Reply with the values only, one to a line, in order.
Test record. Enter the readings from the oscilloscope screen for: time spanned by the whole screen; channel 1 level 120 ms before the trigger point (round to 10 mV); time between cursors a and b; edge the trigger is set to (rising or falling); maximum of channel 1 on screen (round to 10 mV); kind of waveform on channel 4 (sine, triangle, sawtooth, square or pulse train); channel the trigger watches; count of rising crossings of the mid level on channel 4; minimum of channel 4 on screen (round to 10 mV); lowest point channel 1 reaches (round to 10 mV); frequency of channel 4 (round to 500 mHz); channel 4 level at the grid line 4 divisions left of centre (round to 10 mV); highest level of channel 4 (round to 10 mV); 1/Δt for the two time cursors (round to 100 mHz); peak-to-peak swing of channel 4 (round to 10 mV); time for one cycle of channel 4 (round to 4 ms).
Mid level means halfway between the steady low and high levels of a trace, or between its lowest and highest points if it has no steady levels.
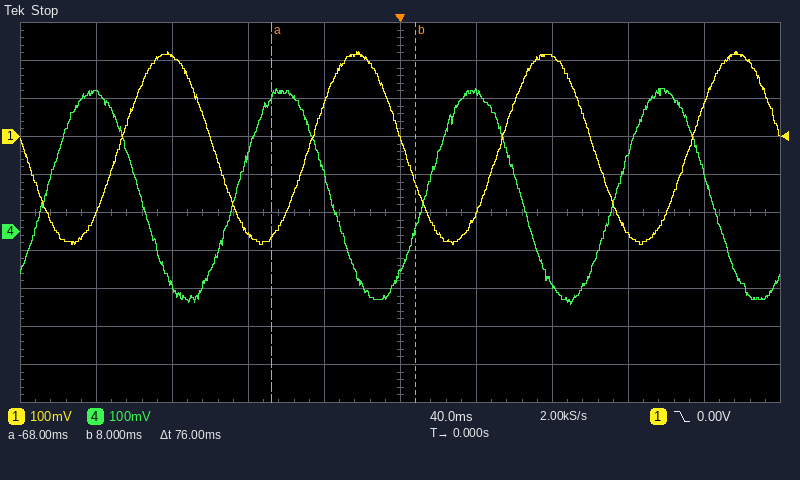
400 ms
210 mV
76 ms
falling
220 mV
sine
channel 1
4
-190 mV
-280 mV
10.0 Hz
360 mV
380 mV
13.2 Hz
570 mV
100 ms
